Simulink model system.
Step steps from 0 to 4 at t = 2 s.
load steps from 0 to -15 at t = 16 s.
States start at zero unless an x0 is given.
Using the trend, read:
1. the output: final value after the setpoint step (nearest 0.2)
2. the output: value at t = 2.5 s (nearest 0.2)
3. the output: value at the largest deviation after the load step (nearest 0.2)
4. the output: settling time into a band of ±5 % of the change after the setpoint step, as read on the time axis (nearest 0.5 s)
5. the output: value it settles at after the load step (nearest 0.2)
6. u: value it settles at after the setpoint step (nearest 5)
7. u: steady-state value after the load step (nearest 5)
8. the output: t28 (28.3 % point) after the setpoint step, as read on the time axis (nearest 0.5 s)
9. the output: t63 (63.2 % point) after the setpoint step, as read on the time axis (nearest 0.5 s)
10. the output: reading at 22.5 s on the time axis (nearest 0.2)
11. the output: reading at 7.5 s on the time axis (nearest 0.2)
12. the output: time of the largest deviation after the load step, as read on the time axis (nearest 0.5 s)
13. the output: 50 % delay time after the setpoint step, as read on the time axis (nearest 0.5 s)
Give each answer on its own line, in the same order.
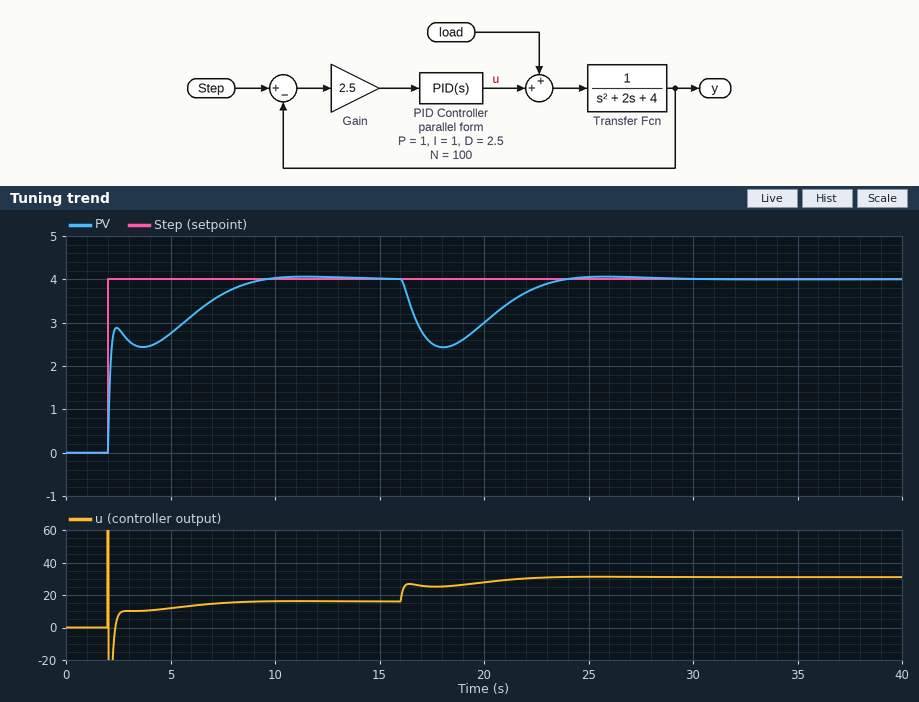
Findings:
4.0
2.8
2.4
8.0 s
4.0
15
30
2.0 s
2.0 s
3.8
3.6
18.0 s
2.0 s
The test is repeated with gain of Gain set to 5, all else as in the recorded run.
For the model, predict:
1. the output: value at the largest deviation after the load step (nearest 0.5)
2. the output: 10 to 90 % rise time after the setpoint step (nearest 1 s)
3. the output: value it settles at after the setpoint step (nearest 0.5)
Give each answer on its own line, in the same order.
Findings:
3.0
4 s
4.0
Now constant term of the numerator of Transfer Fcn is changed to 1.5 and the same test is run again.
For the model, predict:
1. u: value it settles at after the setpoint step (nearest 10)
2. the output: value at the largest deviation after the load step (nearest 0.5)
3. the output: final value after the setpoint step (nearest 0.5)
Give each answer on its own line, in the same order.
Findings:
10
2.0
4.0
